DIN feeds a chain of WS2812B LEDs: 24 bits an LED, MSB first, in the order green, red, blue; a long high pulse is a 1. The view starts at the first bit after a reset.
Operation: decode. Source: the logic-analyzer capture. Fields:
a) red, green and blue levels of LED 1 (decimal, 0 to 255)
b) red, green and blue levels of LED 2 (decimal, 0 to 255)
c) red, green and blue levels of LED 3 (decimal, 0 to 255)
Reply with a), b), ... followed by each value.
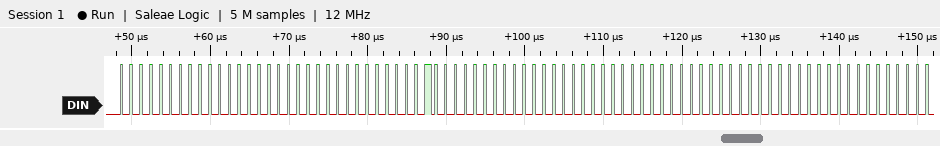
a) 0, 0, 0
b) 0, 1, 0
c) 0, 0, 0
